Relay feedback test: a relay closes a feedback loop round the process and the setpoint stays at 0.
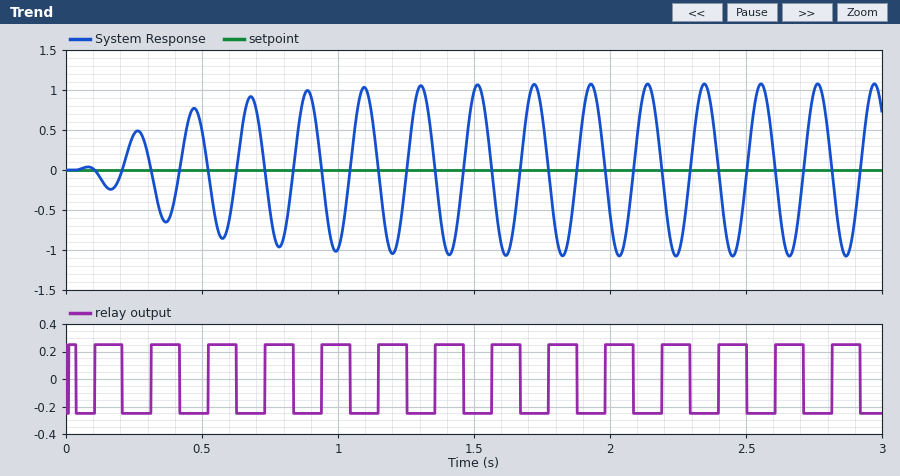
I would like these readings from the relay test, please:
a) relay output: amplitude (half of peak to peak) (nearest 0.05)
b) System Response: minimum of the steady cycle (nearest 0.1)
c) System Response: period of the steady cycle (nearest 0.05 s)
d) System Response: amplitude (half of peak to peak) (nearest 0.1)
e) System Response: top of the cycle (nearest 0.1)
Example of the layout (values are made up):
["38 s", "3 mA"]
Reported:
["0.25", "-1.1", "0.20 s", "1.1", "1.1"]
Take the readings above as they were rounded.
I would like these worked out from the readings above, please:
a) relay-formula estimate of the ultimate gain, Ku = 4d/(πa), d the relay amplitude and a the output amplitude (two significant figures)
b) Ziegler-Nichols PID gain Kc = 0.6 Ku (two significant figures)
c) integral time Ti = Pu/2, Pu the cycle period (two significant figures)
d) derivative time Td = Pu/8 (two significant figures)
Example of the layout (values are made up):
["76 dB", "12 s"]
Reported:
["0.29", "0.17", "0.10 s", "0.025 s"]
